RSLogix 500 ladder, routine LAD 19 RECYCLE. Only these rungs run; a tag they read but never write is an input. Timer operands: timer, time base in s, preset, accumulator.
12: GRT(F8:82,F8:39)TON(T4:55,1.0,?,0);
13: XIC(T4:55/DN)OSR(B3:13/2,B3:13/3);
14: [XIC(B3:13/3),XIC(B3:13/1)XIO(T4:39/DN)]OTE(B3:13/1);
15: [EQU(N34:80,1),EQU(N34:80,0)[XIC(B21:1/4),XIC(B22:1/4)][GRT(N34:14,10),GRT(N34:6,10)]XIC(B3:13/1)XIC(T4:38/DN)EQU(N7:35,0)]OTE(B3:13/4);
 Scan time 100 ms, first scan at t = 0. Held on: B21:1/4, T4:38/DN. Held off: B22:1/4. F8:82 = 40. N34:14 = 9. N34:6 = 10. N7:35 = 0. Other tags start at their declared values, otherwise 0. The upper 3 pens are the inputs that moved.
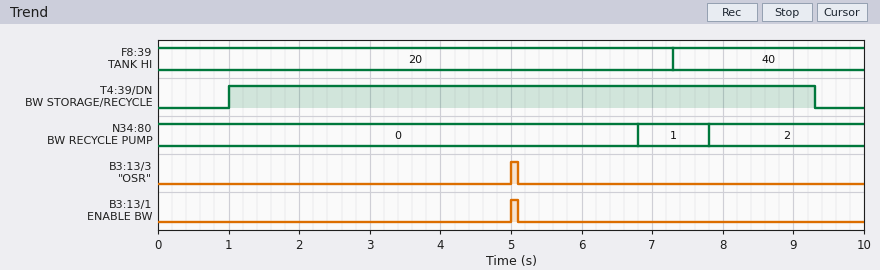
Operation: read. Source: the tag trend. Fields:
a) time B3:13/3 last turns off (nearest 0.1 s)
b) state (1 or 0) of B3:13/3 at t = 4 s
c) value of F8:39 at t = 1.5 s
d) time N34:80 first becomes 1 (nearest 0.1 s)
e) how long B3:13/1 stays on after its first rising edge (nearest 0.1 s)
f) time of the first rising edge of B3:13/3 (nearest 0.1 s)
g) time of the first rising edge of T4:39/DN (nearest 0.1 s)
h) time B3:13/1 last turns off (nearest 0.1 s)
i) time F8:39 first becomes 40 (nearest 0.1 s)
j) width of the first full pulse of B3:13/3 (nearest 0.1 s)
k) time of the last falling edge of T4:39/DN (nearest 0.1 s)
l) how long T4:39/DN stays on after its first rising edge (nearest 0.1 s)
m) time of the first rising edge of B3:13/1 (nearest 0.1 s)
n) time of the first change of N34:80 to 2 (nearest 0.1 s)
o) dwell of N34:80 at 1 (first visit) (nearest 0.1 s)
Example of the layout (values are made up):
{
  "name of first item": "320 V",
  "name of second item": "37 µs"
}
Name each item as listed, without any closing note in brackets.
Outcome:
{
  "time B3:13/3 last turns off": "5.1 s",
  "state (1 or 0) of B3:13/3 at t = 4 s": "0",
  "value of F8:39 at t = 1.5 s": "20",
  "time N34:80 first becomes 1": "6.8 s",
  "how long B3:13/1 stays on after its first rising edge": "0.1 s",
  "time of the first rising edge of B3:13/3": "5.0 s",
  "time of the first rising edge of T4:39/DN": "1.0 s",
  "time B3:13/1 last turns off": "5.1 s",
  "time F8:39 first becomes 40": "7.3 s",
  "width of the first full pulse of B3:13/3": "0.1 s",
  "time of the last falling edge of T4:39/DN": "9.3 s",
  "how long T4:39/DN stays on after its first rising edge": "8.3 s",
  "time of the first rising edge of B3:13/1": "5.0 s",
  "time of the first change of N34:80 to 2": "7.8 s",
  "dwell of N34:80 at 1 (first visit)": "1.0 s"
}
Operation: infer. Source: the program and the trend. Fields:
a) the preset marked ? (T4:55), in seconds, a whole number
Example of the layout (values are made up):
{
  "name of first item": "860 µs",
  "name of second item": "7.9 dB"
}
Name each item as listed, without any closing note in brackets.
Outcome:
{
  "the preset marked ? (T4:55), in seconds, a whole number": "5 s"
}
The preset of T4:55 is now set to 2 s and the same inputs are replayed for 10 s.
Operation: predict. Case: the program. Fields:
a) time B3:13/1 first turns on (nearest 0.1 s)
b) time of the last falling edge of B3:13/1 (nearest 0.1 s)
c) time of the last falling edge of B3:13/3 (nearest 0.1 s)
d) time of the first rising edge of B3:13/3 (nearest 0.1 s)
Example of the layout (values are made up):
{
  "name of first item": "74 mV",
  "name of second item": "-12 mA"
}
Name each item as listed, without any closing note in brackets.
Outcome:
{
  "time B3:13/1 first turns on": "2.0 s",
  "time of the last falling edge of B3:13/1": "2.1 s",
  "time of the last falling edge of B3:13/3": "2.1 s",
  "time of the first rising edge of B3:13/3": "2.0 s"
}
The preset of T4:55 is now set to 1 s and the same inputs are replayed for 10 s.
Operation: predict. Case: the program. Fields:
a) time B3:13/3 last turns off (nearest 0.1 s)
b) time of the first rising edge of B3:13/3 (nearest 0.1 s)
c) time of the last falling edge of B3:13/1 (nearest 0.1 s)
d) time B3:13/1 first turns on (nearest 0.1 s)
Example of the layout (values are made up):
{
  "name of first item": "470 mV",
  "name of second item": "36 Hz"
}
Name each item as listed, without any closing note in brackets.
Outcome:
{
  "time B3:13/3 last turns off": "1.1 s",
  "time of the first rising edge of B3:13/3": "1.0 s",
  "time of the last falling edge of B3:13/1": "1.1 s",
  "time B3:13/1 first turns on": "1.0 s"
}
